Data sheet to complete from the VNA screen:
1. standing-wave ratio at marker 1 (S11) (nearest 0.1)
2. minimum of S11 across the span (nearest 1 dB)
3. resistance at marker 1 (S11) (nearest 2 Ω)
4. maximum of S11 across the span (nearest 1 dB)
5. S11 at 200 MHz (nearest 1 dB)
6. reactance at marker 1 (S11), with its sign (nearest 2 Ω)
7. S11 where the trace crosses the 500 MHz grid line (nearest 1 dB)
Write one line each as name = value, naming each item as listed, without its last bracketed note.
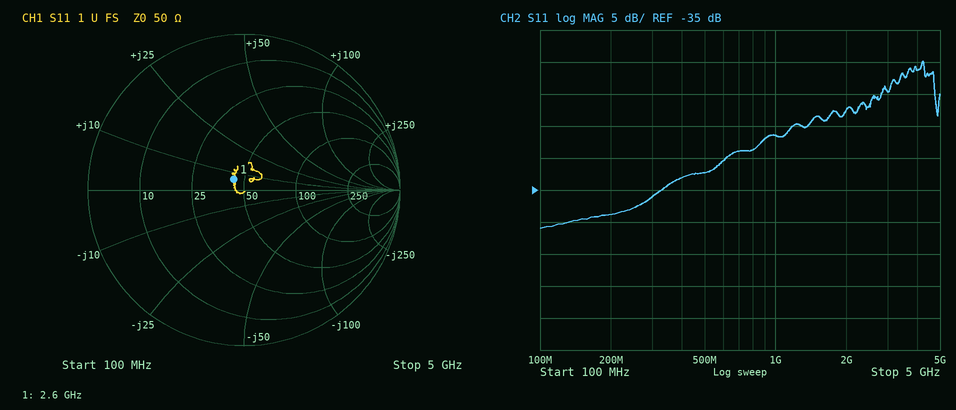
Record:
standing-wave ratio at marker 1 (S11) = 1.2
minimum of S11 across the span = -41 dB
resistance at marker 1 (S11) = 44 Ω
maximum of S11 across the span = -15 dB
S11 at 200 MHz = -39 dB
reactance at marker 1 (S11), with its sign = +6 Ω
S11 where the trace crosses the 500 MHz grid line = -32 dB
